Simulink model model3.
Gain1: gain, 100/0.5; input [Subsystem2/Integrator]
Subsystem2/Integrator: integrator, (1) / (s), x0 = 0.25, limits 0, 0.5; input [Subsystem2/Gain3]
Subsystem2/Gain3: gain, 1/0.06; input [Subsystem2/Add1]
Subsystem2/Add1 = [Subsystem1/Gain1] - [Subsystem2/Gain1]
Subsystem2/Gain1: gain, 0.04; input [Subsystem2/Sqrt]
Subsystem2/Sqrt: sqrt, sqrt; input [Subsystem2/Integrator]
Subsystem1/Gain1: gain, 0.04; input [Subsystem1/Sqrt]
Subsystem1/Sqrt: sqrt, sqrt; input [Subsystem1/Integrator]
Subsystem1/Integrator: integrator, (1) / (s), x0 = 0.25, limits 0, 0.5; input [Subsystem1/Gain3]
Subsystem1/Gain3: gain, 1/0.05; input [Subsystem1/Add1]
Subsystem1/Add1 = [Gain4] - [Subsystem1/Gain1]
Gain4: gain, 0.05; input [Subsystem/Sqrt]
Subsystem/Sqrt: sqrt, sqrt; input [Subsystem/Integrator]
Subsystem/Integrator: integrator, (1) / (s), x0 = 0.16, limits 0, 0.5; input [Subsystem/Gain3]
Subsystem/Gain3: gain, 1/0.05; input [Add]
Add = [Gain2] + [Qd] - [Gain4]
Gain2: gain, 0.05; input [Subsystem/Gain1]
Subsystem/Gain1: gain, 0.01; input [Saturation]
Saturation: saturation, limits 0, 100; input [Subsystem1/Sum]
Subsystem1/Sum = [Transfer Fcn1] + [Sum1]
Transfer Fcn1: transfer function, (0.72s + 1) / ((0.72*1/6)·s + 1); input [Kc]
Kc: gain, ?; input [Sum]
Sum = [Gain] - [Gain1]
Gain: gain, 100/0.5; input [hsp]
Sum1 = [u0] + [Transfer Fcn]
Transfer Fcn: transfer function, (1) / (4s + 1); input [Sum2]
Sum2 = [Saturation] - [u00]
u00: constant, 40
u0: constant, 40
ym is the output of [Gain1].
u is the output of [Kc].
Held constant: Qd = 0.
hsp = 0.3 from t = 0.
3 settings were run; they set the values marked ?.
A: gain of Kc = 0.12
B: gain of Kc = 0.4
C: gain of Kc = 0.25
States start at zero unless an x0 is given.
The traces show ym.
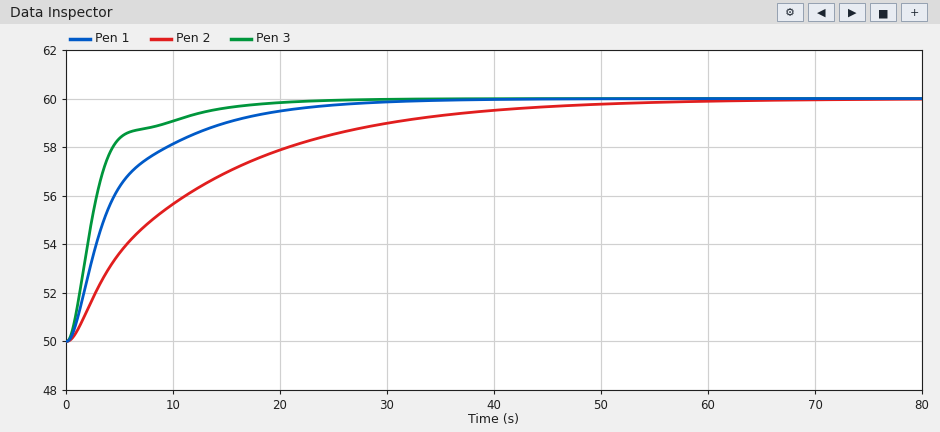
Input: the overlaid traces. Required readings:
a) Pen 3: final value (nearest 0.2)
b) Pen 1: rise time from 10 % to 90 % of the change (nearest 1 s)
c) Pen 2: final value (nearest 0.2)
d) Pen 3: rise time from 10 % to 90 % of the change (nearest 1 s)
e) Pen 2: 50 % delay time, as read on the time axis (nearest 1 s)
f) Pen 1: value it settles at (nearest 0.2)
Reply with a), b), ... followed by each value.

a) 60.0
b) 14 s
c) 60.0
d) 9 s
e) 8 s
f) 60.0
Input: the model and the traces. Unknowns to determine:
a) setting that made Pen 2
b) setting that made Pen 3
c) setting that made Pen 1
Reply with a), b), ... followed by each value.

a) A
b) B
c) C
